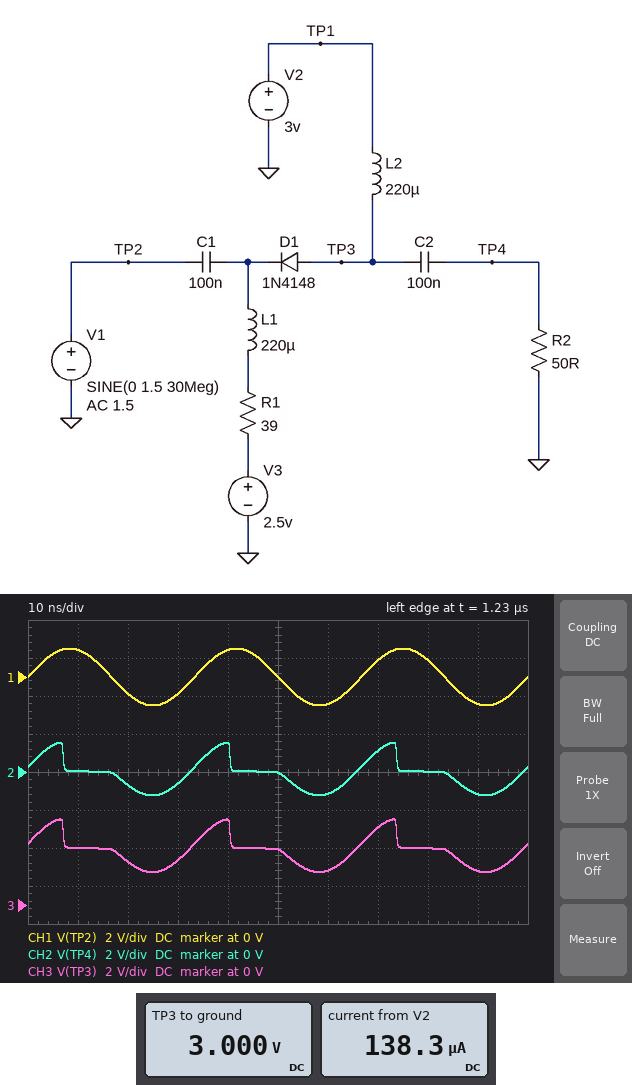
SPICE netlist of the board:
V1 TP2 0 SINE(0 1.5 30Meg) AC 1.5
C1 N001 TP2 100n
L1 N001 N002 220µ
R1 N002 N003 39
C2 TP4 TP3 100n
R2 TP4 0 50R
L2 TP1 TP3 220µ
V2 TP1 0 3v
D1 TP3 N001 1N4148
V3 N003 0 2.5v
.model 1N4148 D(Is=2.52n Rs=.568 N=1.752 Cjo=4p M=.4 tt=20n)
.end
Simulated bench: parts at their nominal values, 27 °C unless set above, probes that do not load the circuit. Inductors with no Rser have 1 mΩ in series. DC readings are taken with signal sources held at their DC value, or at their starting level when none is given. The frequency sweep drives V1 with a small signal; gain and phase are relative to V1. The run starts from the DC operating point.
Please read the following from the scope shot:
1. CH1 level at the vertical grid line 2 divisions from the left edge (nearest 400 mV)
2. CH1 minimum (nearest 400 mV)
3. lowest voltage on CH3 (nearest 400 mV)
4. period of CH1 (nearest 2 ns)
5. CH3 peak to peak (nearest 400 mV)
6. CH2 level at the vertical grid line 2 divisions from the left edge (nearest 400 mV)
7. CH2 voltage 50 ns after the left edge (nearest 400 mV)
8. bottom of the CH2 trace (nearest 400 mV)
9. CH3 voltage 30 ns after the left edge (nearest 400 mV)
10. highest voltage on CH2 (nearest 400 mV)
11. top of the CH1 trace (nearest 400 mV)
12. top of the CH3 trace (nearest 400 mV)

-800 mV
-1.6 V
1.6 V
34 ns
2.8 V
-800 mV
0 V
-1.2 V
2.4 V
1.6 V
1.6 V
4.4 V
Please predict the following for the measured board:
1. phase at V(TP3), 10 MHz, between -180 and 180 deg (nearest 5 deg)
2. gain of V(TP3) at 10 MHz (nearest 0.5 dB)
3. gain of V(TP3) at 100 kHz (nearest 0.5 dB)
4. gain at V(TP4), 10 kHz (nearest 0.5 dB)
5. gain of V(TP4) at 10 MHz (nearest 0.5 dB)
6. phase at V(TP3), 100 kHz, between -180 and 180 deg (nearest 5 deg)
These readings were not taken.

45 deg
-13.0 dB
-16.0 dB
-49.5 dB
-13.0 dB
10 deg
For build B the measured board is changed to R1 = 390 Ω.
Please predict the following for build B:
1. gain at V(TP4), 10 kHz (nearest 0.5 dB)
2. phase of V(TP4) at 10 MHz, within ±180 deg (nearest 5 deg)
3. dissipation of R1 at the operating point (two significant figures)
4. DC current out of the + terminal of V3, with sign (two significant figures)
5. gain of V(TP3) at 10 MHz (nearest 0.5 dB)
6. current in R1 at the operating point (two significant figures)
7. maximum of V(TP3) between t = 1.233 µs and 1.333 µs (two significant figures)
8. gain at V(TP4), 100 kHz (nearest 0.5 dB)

-43.5 dB
50 deg
2.4 µW
-79 µA
-17.0 dB
79 µA
4.5 V
-21.5 dB
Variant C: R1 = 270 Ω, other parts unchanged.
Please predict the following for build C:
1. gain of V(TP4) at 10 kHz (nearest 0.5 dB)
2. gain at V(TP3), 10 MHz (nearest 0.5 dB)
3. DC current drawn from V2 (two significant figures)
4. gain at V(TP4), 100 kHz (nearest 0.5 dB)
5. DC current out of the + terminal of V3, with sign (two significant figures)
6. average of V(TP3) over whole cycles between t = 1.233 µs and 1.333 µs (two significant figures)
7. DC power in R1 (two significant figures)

-43.5 dB
-16.0 dB
91 µA
-20.5 dB
-91 µA
2.8 V
2.2 µW
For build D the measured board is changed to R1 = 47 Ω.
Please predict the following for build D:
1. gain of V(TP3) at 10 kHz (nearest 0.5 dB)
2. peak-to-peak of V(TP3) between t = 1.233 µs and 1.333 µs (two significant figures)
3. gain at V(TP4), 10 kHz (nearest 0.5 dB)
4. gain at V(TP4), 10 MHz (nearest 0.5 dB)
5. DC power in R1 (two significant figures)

-38.0 dB
2.8 V
-48.5 dB
-13.5 dB
860 nW
